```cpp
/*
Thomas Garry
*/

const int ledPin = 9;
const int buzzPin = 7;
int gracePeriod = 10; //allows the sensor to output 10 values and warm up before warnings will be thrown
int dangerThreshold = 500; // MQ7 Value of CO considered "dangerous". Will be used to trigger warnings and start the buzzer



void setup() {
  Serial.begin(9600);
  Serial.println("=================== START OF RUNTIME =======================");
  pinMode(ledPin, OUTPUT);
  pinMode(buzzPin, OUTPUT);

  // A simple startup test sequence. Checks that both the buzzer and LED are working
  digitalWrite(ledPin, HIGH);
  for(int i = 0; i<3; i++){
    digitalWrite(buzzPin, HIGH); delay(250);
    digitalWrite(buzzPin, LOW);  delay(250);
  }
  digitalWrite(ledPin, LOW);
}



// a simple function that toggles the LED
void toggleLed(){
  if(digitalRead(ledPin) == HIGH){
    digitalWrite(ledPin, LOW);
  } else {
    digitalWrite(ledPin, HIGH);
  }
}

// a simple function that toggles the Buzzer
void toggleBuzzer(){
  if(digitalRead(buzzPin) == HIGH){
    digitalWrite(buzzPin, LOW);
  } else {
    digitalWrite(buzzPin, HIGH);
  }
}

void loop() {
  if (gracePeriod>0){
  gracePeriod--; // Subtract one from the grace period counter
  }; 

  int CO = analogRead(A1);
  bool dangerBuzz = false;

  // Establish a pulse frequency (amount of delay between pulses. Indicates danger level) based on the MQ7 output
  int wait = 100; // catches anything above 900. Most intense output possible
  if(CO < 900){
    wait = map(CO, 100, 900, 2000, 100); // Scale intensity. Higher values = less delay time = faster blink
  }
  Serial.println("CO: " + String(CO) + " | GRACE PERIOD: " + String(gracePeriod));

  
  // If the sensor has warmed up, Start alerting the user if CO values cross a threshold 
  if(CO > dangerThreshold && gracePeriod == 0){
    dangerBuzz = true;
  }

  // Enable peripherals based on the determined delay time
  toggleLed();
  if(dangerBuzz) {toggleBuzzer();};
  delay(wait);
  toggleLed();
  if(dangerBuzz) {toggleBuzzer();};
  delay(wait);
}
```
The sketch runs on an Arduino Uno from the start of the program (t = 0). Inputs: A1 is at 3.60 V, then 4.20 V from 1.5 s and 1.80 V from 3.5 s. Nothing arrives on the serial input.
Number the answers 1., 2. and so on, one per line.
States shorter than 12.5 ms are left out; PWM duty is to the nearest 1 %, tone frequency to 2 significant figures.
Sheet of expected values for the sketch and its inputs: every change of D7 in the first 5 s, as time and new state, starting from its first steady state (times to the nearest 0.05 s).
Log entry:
1. 0 s high; 0.25 s low; 0.5 s high; 0.75 s low; 1 s high; 1.25 s low
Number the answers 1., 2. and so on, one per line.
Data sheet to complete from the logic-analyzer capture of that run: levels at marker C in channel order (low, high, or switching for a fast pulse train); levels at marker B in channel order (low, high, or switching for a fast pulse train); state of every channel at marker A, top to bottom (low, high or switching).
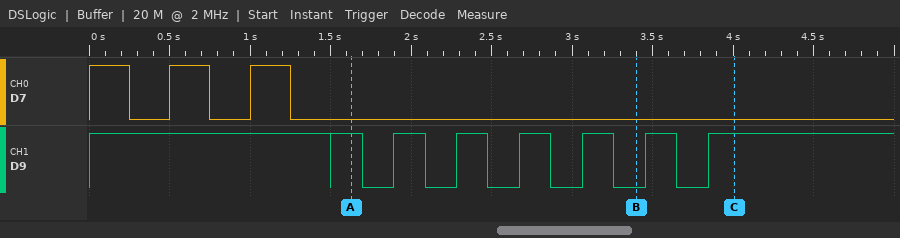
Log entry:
1. D7 low, D9 high
2. D7 low, D9 low
3. D7 low, D9 high
